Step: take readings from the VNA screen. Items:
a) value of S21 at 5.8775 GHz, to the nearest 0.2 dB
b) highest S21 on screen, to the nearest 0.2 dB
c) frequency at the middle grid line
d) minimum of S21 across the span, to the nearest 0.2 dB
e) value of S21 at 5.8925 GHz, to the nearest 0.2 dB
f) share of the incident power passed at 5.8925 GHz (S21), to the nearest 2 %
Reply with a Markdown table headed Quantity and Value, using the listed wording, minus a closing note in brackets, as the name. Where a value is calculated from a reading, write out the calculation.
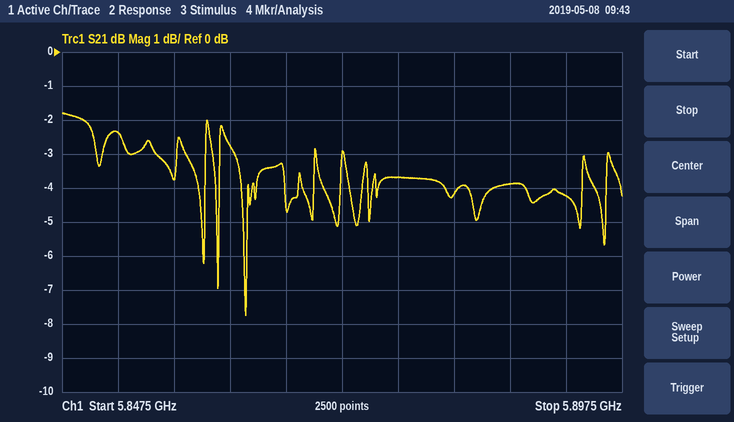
| Quantity | Value |
|---|---|
| value of S21 at 5.8775 GHz, to the nearest 0.2 dB | -3.6 dB |
| highest S21 on screen, to the nearest 0.2 dB | -1.8 dB |
| frequency at the middle grid line | 5.8725 GHz |
| minimum of S21 across the span, to the nearest 0.2 dB | -7.8 dB |
| value of S21 at 5.8925 GHz, to the nearest 0.2 dB | -4.2 dB |
| share of the incident power passed at 5.8925 GHz (S21), to the nearest 2 % | 10^(-4.2/10) ≈ 38 % |
